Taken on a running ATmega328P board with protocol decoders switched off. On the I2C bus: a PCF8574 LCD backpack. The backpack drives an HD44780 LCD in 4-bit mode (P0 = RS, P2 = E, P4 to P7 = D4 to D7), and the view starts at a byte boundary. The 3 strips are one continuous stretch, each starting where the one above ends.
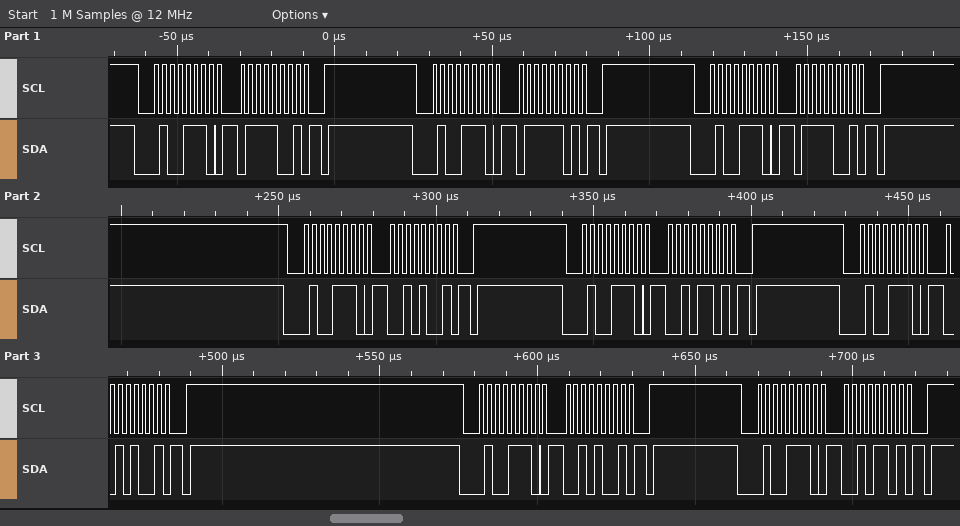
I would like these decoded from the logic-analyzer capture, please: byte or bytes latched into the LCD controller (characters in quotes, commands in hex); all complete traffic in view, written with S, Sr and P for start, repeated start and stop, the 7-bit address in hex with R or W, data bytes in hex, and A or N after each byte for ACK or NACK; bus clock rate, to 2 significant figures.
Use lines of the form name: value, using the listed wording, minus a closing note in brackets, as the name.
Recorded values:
byte or bytes latched into the LCD controller: 'r'
all complete traffic in view, written with S, Sr and P for start, repeated start and stop, the 7-bit address in hex with R or W, data bytes in hex, and A or N after each byte for ACK or NACK: S 27W A 79 A P S 27W A 7D A P S 27W A 79 A P S 27W A 29 A P S 27W A 2D A P S 27W A 29 A P S 27W A 29 A P S 27W A 2D A P
bus clock rate, to 2 significant figures: 400 kHz
